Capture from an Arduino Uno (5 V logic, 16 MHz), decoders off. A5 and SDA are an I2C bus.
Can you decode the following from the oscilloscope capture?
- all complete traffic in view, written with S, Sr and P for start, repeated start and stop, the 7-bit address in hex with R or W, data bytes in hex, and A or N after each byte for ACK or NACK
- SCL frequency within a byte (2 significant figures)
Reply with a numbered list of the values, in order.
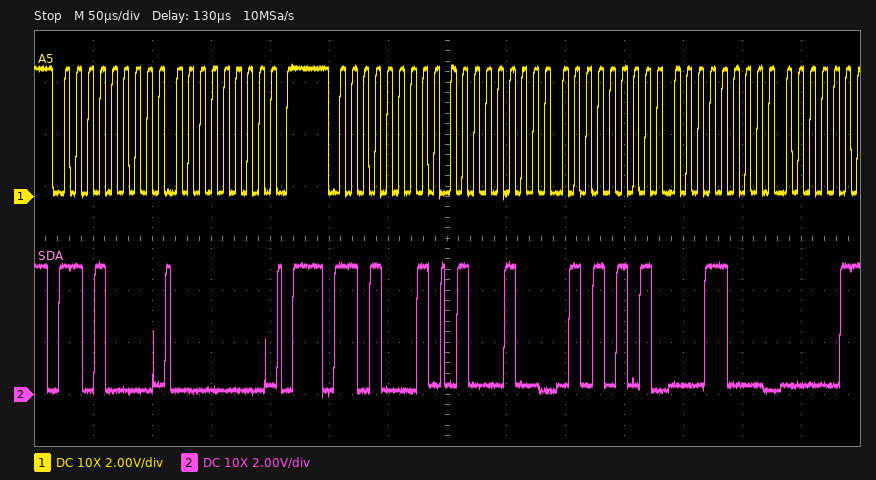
1. S 68W A 00 A P S 68R A 44 A 55 A 18 A
2. 100 kHz
